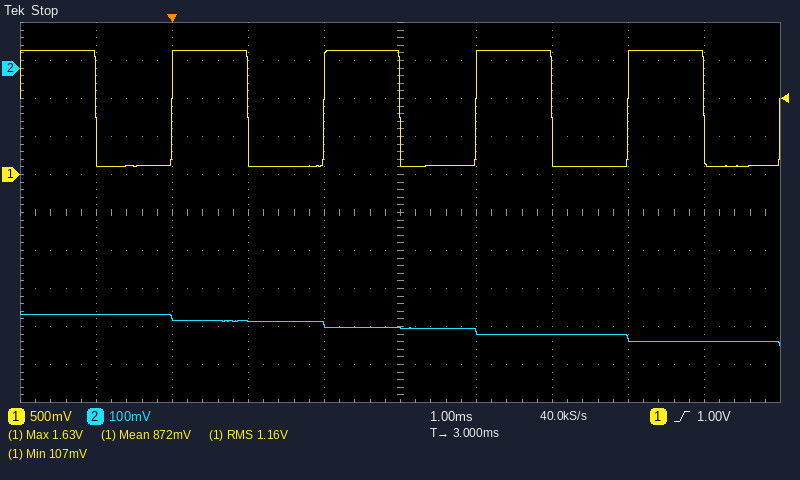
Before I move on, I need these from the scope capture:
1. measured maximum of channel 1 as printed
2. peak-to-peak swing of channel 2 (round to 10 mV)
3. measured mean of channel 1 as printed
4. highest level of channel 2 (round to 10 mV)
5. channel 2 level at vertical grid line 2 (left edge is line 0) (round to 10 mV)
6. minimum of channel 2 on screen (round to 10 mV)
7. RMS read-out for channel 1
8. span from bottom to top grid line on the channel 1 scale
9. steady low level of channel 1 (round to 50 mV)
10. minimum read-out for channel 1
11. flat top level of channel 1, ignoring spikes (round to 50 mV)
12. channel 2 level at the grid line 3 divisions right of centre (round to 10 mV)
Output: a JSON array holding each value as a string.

["1.63 V", "90 mV", "872 mV", "-640 mV", "-660 mV", "-730 mV", "1.16 V", "5 V", "100 mV", "107 mV", "1.65 V", "-710 mV"]
